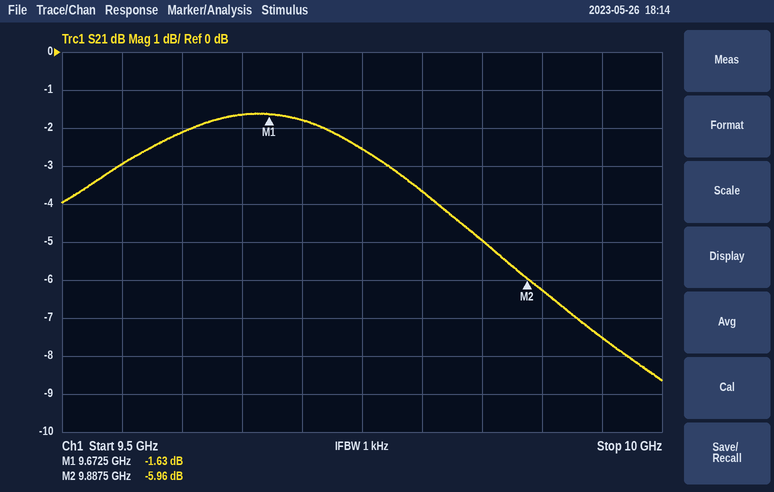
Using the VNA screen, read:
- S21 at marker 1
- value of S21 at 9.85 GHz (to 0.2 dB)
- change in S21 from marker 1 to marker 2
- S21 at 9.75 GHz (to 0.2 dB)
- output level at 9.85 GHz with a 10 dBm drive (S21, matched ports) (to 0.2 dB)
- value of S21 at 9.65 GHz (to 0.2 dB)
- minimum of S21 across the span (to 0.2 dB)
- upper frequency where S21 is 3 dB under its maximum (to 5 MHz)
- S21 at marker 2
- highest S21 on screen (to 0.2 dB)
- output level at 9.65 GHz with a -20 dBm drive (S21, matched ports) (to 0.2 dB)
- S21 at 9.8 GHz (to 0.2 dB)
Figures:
-1.63 dB
-5.0 dB
-4.33 dB
-2.6 dB
5.0 dBm
-1.6 dB
-8.6 dB
9.835 GHz
-5.96 dB
-1.6 dB
-21.6 dBm
-3.6 dB
